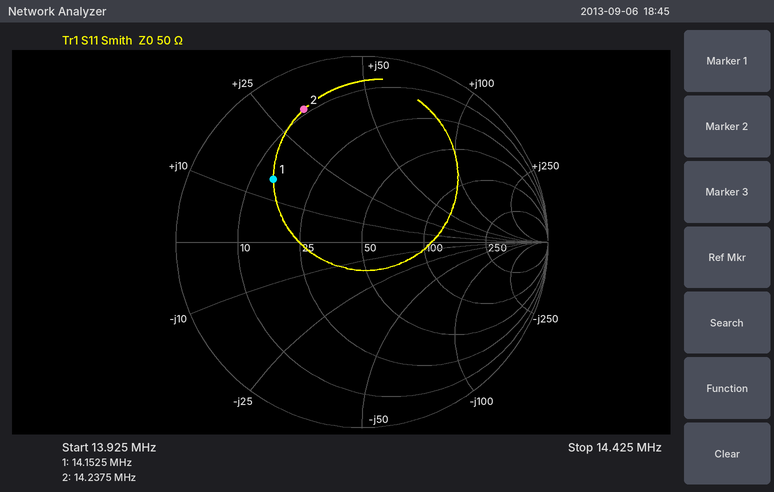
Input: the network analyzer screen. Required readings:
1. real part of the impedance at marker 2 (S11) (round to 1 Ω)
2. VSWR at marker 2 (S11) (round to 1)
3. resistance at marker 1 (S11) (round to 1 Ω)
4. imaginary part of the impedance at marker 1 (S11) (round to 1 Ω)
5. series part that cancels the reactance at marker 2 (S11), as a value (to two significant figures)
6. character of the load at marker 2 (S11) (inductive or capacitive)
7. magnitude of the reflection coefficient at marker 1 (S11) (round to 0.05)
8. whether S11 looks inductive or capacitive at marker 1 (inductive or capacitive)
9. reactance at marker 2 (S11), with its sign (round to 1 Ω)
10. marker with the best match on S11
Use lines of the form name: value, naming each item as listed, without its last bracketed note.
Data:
real part of the impedance at marker 2 (S11): 9 Ω
VSWR at marker 2 (S11): 8
resistance at marker 1 (S11): 14 Ω
imaginary part of the impedance at marker 1 (S11): +15 Ω
series part that cancels the reactance at marker 2 (S11), as a value: 350 pF
character of the load at marker 2 (S11): inductive
magnitude of the reflection coefficient at marker 1 (S11): 0.60
whether S11 looks inductive or capacitive at marker 1: inductive
reactance at marker 2 (S11), with its sign: +32 Ω
marker with the best match on S11: marker 1
